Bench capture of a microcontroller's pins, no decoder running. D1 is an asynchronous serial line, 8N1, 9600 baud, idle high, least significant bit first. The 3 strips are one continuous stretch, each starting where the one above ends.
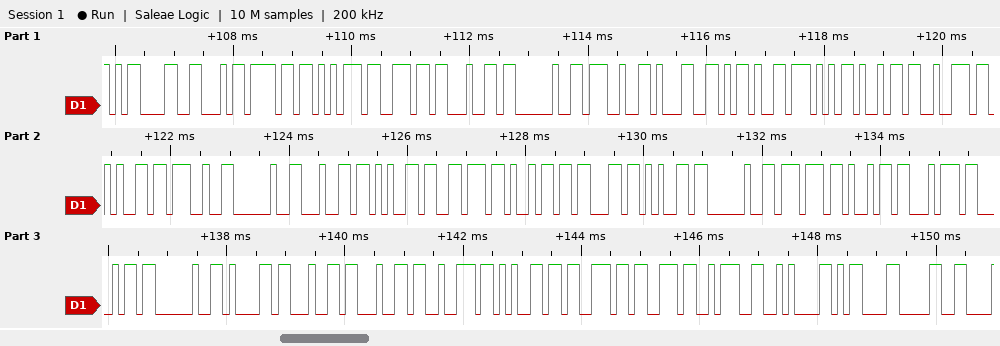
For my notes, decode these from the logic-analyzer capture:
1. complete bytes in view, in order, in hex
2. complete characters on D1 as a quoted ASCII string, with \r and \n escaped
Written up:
0D 46 6F 75 6E 64 20 27 31 2D 57 69 72 65 27 20 64 65 76 69 63 65 20 77 69 74 68 20 61 64 64 72 65 73 73 3A 0A 0D 30
"\rFound '1-Wire' device with address:\n\r0"
